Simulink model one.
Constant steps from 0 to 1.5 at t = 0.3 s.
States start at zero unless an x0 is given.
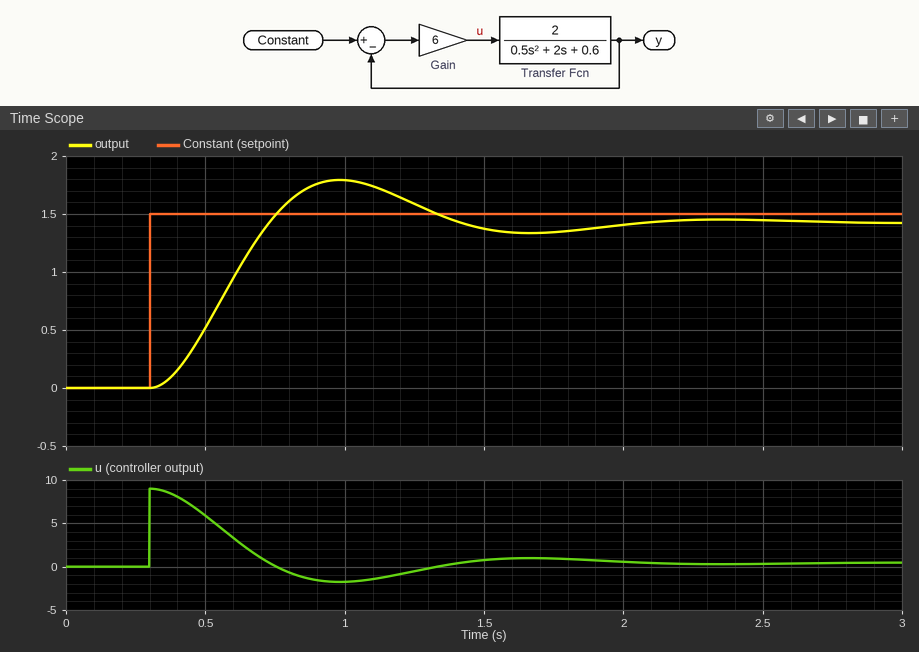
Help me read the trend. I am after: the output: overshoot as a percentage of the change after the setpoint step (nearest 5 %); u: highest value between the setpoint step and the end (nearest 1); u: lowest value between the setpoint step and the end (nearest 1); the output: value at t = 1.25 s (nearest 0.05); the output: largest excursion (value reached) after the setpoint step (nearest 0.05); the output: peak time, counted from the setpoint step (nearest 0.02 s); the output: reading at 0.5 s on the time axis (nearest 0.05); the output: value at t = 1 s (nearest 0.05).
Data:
25 %
9
-2
1.60
1.80
0.68 s
0.50
1.80
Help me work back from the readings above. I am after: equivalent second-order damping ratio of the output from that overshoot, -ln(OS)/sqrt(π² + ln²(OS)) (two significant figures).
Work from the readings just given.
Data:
0.40
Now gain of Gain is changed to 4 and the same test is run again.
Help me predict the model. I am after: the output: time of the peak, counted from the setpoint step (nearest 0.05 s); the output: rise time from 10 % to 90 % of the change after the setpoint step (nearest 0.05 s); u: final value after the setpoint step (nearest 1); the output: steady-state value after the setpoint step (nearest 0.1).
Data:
0.85 s
0.40 s
0
1.4
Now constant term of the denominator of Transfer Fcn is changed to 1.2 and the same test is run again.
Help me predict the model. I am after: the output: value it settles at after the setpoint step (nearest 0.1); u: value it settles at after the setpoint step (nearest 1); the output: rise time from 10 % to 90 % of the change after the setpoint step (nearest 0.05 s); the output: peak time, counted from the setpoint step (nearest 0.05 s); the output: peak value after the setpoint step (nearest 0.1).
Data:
1.4
1
0.30 s
0.65 s
1.7
